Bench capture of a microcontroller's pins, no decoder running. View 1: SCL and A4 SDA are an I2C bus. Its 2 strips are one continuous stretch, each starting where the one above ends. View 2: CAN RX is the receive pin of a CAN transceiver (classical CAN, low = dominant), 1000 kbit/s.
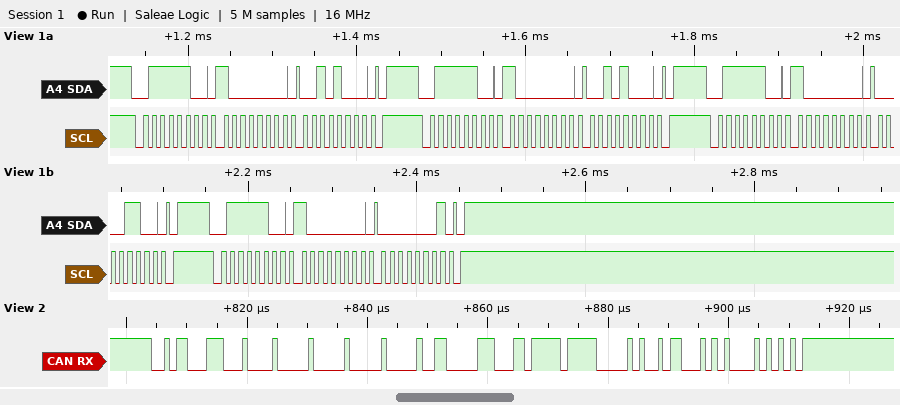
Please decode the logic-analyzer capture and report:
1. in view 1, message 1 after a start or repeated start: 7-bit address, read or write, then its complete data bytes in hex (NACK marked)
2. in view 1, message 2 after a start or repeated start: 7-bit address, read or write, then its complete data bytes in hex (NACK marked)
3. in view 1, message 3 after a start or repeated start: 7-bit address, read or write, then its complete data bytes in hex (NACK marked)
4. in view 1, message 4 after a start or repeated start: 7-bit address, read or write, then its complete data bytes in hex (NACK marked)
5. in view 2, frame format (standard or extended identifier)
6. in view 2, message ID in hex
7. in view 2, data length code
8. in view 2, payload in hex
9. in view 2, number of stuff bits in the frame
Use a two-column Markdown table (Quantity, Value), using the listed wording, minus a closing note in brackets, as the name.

| Quantity | Value |
|---|---|
| in view 1, message 1 after a start or repeated start: 7-bit address, read or write, then its complete data bytes in hex | 0x3E write: 80 28 |
| in view 1, message 2 after a start or repeated start: 7-bit address, read or write, then its complete data bytes in hex | 0x3E write: 80 28 |
| in view 1, message 3 after a start or repeated start: 7-bit address, read or write, then its complete data bytes in hex | 0x3E write: 80 0C |
| in view 1, message 4 after a start or repeated start: 7-bit address, read or write, then its complete data bytes in hex | 0x3E write: 80 01 |
| in view 2, frame format | standard |
| in view 2, message ID in hex | 0x2C7 |
| in view 2, data length code | 8 |
| in view 2, payload in hex | 40 00 00 C1 8D FF 82 58 |
| in view 2, number of stuff bits in the frame | 8 |
